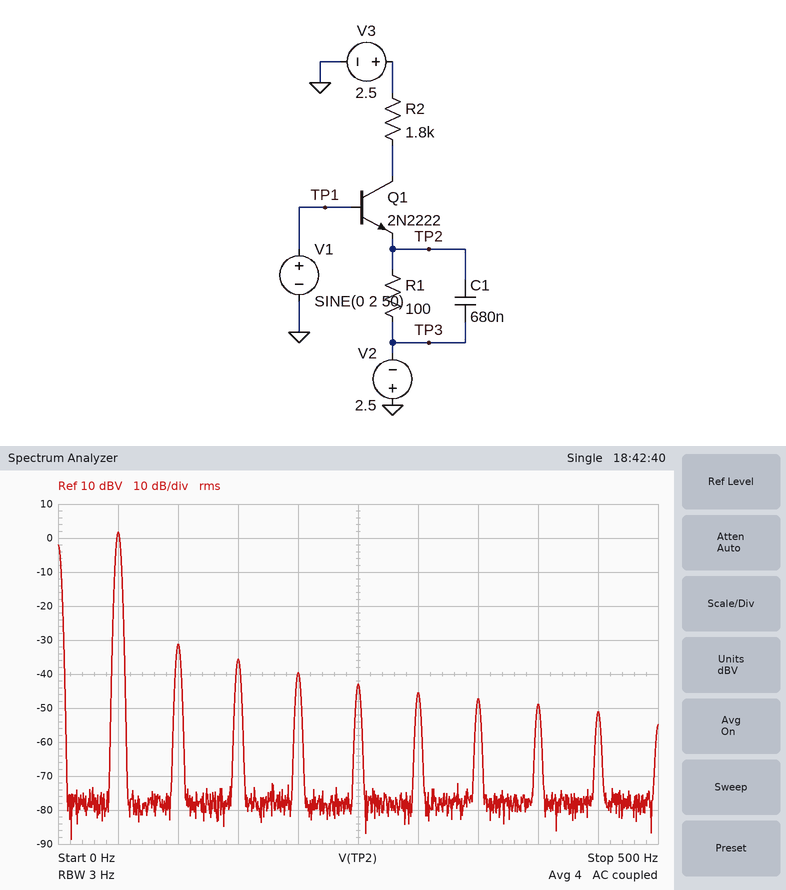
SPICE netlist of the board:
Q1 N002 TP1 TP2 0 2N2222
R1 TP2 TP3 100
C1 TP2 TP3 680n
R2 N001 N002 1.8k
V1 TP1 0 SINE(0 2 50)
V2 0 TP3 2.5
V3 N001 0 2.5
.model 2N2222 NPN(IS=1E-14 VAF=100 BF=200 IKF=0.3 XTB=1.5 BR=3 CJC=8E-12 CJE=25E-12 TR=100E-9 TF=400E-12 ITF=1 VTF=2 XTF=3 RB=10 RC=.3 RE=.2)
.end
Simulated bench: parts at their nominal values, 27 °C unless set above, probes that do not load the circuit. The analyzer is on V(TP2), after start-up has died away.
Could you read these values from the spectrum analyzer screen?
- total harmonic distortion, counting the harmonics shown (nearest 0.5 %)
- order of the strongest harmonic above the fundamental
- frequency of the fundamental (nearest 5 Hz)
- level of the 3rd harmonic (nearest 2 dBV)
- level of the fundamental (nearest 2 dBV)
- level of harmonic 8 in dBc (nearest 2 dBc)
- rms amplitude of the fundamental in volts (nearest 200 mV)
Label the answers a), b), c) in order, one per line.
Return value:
a) 3.0 %
b) 2
c) 50 Hz
d) -36 dBV
e) 2 dBV
f) -50 dBc
g) 1.2 V
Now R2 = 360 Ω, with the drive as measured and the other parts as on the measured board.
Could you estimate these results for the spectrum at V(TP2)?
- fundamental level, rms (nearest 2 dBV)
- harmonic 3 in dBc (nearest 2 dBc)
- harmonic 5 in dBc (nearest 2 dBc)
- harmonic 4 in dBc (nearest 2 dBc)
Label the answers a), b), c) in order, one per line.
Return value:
a) 2 dBV
b) -44 dBc
c) -38 dBc
d) -38 dBc
